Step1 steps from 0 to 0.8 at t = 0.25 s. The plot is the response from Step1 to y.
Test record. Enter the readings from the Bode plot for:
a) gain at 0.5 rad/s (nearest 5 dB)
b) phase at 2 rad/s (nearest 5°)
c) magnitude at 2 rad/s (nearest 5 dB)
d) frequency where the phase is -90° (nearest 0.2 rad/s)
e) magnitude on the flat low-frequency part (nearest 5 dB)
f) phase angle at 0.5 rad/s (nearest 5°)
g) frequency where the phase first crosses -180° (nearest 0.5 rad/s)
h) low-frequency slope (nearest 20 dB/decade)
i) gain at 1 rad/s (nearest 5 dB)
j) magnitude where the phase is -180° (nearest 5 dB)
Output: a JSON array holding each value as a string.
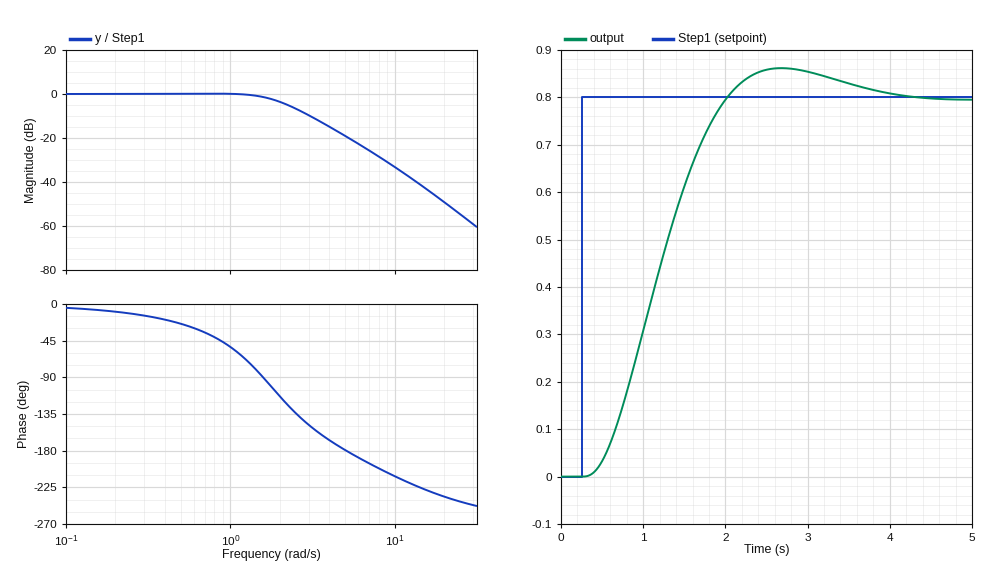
["0 dB", "-115°", "-5 dB", "1.6 rad/s", "0 dB", "-25°", "5.0 rad/s", "0 dB/decade", "0 dB", "-20 dB"]
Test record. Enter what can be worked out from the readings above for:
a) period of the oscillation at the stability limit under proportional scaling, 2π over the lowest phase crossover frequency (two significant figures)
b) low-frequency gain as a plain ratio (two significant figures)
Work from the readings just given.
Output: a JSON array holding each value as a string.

["1.3 s", "1.0"]
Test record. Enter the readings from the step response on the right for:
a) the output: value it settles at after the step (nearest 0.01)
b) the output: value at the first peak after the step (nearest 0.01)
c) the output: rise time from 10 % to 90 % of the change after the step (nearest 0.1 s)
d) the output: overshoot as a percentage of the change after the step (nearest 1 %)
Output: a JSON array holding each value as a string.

["0.80", "0.86", "1.1 s", "8 %"]
